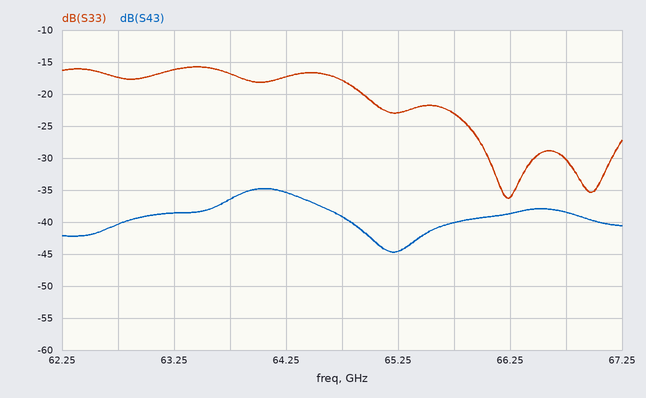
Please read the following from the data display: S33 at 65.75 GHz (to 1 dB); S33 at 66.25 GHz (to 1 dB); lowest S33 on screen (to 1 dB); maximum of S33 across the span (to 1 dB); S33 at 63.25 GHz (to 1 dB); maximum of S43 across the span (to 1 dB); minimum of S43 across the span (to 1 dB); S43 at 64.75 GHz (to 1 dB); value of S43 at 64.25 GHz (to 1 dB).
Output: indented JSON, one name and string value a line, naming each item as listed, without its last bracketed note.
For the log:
{
  "S33 at 65.75 GHz": "-23 dB",
  "S33 at 66.25 GHz": "-36 dB",
  "lowest S33 on screen": "-36 dB",
  "maximum of S33 across the span": "-16 dB",
  "S33 at 63.25 GHz": "-16 dB",
  "maximum of S43 across the span": "-35 dB",
  "minimum of S43 across the span": "-45 dB",
  "S43 at 64.75 GHz": "-39 dB",
  "value of S43 at 64.25 GHz": "-35 dB"
}
